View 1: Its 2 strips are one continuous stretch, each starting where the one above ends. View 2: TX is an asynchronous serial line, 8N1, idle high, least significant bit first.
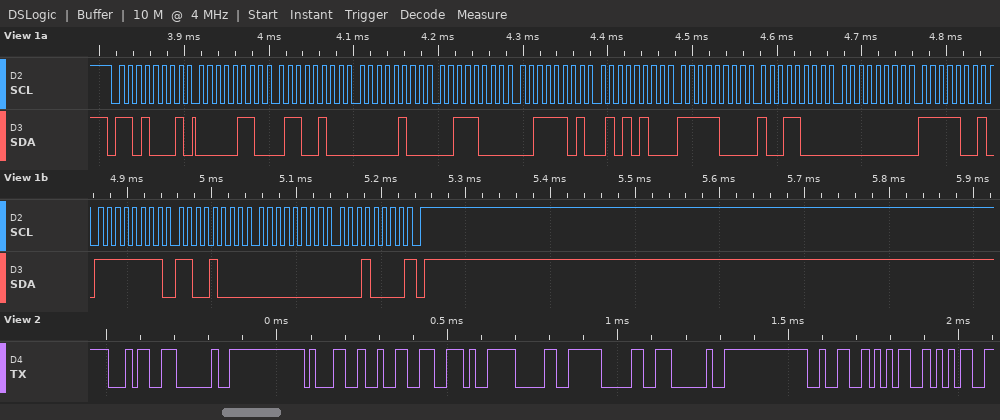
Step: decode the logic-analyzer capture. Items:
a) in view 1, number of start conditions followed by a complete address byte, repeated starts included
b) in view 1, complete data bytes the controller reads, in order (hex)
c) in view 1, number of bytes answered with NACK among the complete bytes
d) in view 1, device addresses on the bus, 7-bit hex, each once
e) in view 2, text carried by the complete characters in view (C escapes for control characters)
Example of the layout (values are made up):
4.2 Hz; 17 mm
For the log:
1; 06 64 04 38 3D 54 F8 98 00 F9 FF C8 00 10; 1; 0x68; "4 12.00 255"
